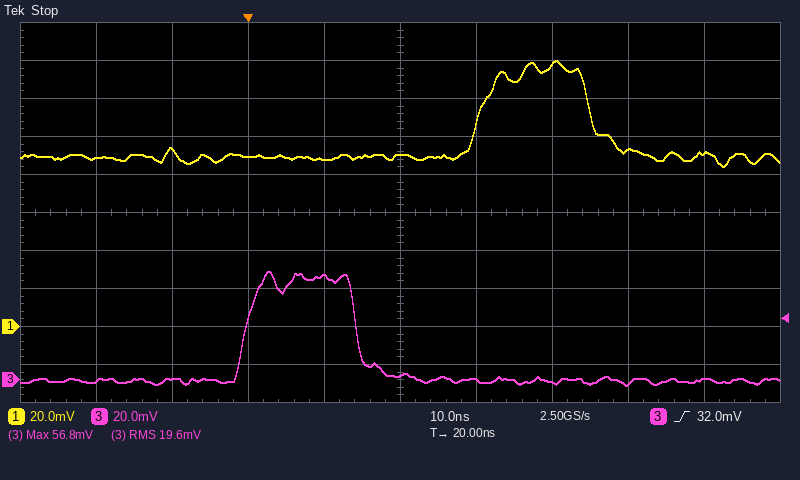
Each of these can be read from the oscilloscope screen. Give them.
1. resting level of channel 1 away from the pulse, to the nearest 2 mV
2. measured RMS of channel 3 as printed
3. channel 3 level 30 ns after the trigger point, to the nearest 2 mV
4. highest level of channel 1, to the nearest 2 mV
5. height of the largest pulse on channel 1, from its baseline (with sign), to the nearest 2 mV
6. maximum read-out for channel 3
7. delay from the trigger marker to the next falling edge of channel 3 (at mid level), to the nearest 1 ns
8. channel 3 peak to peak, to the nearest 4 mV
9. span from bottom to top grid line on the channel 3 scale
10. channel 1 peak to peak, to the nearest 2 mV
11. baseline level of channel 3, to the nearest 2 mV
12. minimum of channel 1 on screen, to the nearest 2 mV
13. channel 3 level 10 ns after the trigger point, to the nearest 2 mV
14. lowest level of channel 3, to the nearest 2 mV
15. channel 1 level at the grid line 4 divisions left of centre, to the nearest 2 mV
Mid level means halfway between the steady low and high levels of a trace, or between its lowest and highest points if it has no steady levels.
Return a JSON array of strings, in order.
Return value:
["90 mV", "19.6 mV", "0 mV", "140 mV", "+50 mV", "56.8 mV", "14 ns", "60 mV", "200 mV", "56 mV", "0 mV", "84 mV", "54 mV", "-4 mV", "88 mV"]
